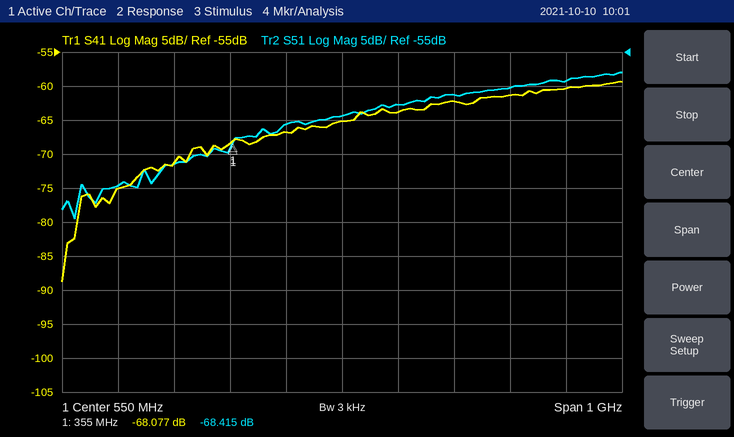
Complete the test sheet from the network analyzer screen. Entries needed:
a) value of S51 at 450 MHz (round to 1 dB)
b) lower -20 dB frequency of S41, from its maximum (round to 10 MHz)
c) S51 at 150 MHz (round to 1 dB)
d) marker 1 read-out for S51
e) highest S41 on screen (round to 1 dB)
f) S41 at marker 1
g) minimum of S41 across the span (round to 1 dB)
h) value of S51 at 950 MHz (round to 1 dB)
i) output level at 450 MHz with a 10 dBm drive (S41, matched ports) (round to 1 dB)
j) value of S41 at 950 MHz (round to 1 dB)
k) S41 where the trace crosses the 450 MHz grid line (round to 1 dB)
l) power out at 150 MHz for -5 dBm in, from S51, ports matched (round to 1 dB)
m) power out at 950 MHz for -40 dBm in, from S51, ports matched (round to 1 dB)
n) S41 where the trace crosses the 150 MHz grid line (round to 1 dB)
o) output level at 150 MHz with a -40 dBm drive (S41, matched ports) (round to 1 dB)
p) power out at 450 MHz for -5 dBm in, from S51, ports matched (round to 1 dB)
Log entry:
-66 dB
80 MHz
-75 dB
-68.415 dB
-59 dB
-68.077 dB
-89 dB
-59 dB
-57 dBm
-60 dB
-67 dB
-80 dBm
-99 dBm
-75 dB
-115 dBm
-71 dBm
